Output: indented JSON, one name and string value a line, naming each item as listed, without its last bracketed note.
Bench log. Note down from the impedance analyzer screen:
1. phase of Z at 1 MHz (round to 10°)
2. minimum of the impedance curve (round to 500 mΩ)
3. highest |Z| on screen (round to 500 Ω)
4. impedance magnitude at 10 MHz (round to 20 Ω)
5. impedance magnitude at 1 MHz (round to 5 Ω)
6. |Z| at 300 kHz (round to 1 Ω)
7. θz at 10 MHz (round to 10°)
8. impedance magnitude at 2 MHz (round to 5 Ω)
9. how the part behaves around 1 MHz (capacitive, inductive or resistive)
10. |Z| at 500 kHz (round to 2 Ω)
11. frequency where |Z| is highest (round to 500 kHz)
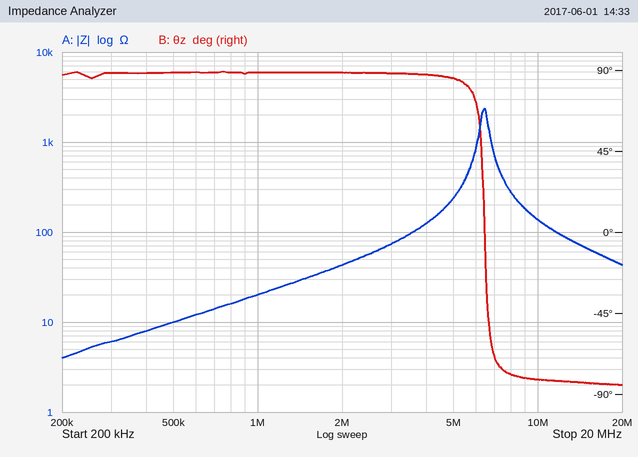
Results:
{
  "phase of Z at 1 MHz": "90°",
  "minimum of the impedance curve": "4.0 Ω",
  "highest |Z| on screen": "2.5 kΩ",
  "impedance magnitude at 10 MHz": "140 Ω",
  "impedance magnitude at 1 MHz": "20 Ω",
  "|Z| at 300 kHz": "6 Ω",
  "θz at 10 MHz": "-80°",
  "impedance magnitude at 2 MHz": "45 Ω",
  "how the part behaves around 1 MHz": "inductive",
  "|Z| at 500 kHz": "10 Ω",
  "frequency where |Z| is highest": "6.5 MHz"
}
